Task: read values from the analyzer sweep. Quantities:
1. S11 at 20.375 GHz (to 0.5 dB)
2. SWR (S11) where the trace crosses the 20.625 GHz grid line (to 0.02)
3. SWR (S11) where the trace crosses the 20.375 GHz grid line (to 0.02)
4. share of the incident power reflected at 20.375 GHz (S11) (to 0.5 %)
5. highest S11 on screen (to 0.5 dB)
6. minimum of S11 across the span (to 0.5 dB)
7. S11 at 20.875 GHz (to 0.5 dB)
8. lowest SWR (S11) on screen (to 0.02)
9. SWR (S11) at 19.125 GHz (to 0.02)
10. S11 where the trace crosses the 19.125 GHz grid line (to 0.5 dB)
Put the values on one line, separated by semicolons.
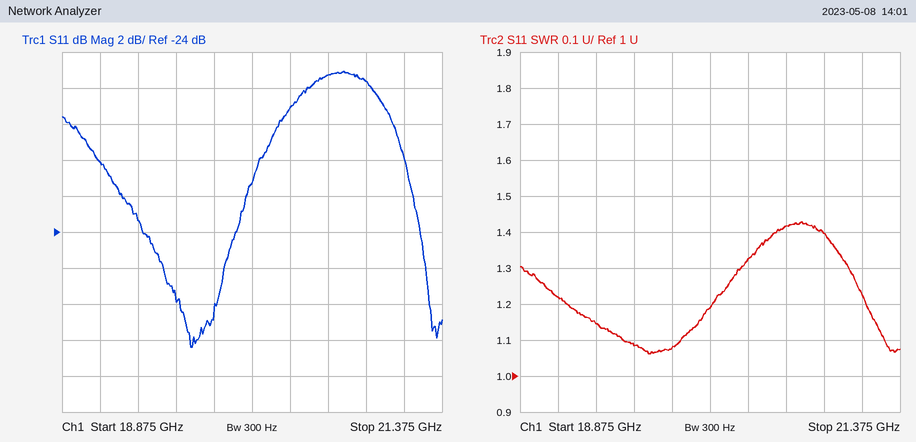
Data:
-17.0 dB; 1.42; 1.32; 2.0 %; -15.0 dB; -30.5 dB; -15.5 dB; 1.06; 1.22; -20.0 dB
